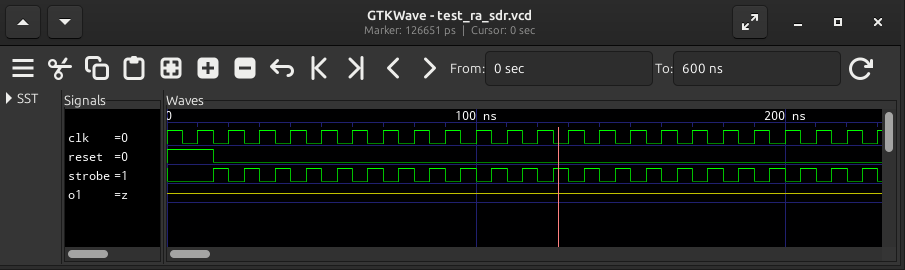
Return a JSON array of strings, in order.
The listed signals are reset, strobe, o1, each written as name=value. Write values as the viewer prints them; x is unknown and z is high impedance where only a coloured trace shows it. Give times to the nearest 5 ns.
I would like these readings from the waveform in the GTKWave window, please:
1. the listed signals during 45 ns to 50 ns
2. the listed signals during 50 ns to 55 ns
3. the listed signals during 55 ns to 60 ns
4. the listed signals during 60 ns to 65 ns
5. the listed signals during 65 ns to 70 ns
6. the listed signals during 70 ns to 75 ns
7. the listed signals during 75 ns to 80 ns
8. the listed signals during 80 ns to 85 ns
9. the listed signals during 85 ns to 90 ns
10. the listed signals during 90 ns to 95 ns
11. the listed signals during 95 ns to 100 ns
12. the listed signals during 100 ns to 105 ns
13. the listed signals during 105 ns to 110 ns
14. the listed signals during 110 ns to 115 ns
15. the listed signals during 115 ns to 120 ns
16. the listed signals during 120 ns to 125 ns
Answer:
["reset=0, strobe=1, o1=z", "reset=0, strobe=0, o1=z", "reset=0, strobe=1, o1=z", "reset=0, strobe=0, o1=z", "reset=0, strobe=1, o1=z", "reset=0, strobe=0, o1=z", "reset=0, strobe=1, o1=z", "reset=0, strobe=0, o1=z", "reset=0, strobe=1, o1=z", "reset=0, strobe=0, o1=z", "reset=0, strobe=1, o1=z", "reset=0, strobe=0, o1=z", "reset=0, strobe=1, o1=z", "reset=0, strobe=0, o1=z", "reset=0, strobe=1, o1=z", "reset=0, strobe=0, o1=z"]
